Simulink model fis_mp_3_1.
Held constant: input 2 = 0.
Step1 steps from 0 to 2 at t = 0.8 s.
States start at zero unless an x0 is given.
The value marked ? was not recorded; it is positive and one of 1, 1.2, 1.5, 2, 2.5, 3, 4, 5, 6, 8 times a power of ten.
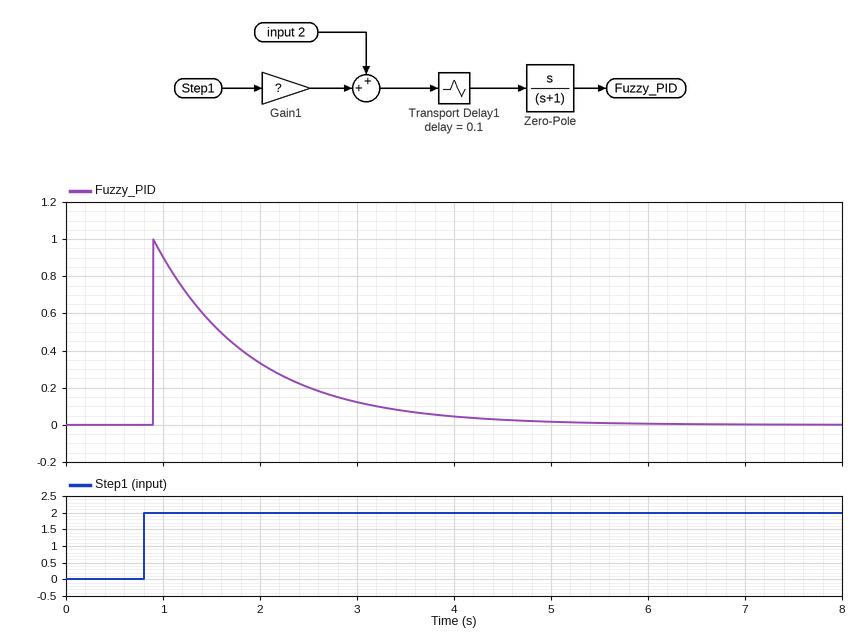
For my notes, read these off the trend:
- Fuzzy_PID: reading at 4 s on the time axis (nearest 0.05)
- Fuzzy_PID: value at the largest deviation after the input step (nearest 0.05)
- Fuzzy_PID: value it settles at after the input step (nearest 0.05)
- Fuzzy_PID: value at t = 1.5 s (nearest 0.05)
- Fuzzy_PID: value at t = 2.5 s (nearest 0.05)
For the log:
0.05
1.00
0.00
0.55
0.20
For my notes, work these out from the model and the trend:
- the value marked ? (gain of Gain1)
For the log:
0.5
